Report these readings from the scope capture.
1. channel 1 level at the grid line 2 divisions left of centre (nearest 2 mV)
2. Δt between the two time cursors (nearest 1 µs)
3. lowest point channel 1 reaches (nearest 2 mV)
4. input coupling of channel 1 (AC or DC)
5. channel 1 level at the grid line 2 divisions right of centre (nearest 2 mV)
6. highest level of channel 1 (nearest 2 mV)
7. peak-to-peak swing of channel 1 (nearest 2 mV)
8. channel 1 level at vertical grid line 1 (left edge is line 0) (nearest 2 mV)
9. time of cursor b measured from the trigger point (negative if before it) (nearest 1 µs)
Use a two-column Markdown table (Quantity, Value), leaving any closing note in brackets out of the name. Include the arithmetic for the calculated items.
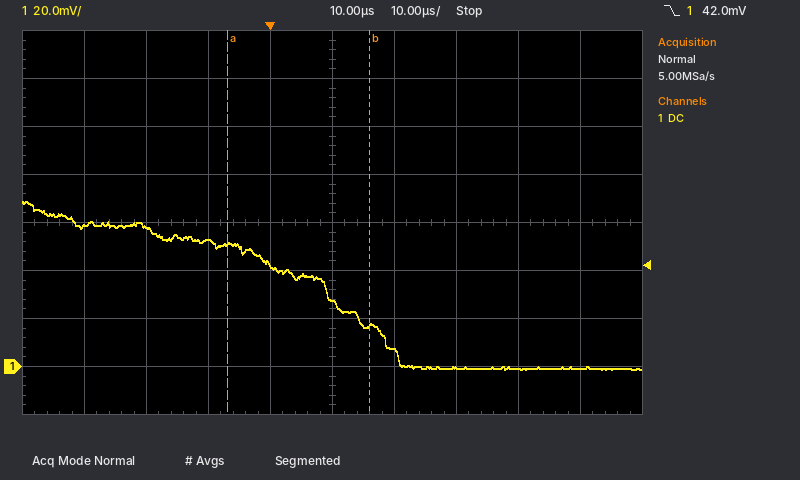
| Quantity | Value |
|---|---|
| channel 1 level at the grid line 2 divisions left of centre | 52 mV |
| Δt between the two time cursors | 23 µs |
| lowest point channel 1 reaches | -2 mV |
| input coupling of channel 1 | DC |
| channel 1 level at the grid line 2 divisions right of centre | 0 mV |
| highest level of channel 1 | 68 mV |
| peak-to-peak swing of channel 1 | 68 mV − (-2 mV) = 70 mV |
| channel 1 level at vertical grid line 1 (left edge is line 0) | 58 mV |
| time of cursor b measured from the trigger point (negative if before it) | +16 µs |
